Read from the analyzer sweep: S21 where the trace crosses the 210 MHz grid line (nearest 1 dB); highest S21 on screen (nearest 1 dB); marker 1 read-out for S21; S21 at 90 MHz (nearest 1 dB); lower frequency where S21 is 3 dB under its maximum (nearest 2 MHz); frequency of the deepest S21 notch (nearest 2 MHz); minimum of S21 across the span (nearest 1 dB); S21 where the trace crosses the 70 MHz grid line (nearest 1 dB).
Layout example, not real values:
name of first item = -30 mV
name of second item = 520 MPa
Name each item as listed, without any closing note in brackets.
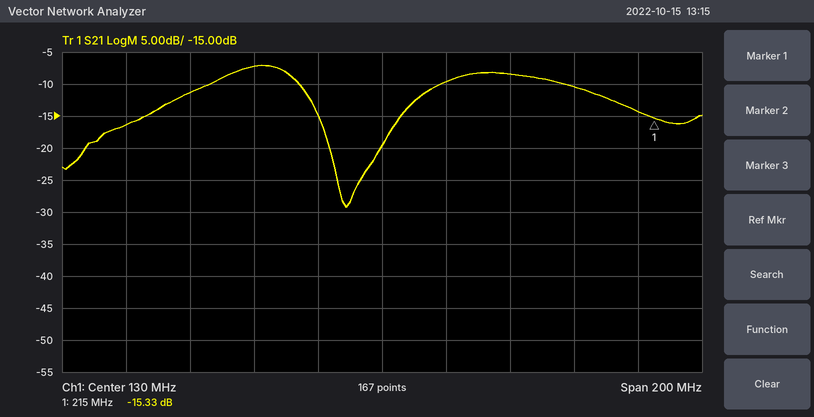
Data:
S21 where the trace crosses the 210 MHz grid line = -14 dB
highest S21 on screen = -7 dB
marker 1 read-out for S21 = -15.33 dB
S21 at 90 MHz = -7 dB
lower frequency where S21 is 3 dB under its maximum = 76 MHz
frequency of the deepest S21 notch = 118 MHz
minimum of S21 across the span = -29 dB
S21 where the trace crosses the 70 MHz grid line = -11 dB
